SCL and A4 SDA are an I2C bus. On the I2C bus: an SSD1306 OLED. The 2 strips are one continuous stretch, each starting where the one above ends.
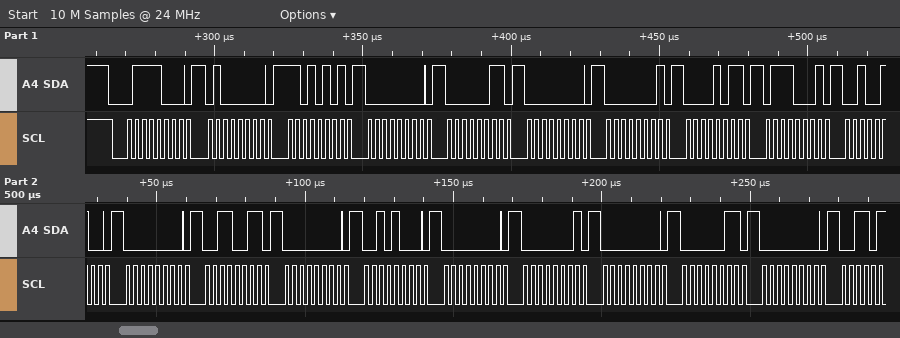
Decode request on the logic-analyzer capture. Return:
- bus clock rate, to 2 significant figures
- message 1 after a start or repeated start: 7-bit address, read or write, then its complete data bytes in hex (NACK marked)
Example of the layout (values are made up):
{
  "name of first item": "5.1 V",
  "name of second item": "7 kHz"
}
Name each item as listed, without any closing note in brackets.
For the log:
{
  "bus clock rate, to 2 significant figures": "400 kHz",
  "message 1 after a start or repeated start: 7-bit address, read or write, then its complete data bytes in hex": "0x3C write: 40 D5 00 03 00 01 0B 71 24 00 33 00 28 00 01 00 03 00"
}
